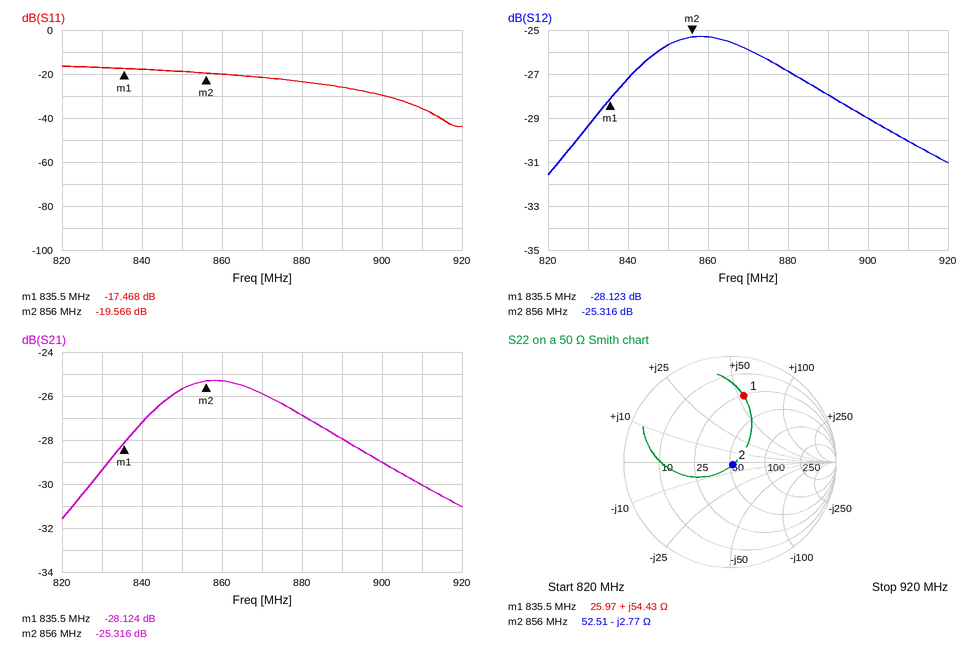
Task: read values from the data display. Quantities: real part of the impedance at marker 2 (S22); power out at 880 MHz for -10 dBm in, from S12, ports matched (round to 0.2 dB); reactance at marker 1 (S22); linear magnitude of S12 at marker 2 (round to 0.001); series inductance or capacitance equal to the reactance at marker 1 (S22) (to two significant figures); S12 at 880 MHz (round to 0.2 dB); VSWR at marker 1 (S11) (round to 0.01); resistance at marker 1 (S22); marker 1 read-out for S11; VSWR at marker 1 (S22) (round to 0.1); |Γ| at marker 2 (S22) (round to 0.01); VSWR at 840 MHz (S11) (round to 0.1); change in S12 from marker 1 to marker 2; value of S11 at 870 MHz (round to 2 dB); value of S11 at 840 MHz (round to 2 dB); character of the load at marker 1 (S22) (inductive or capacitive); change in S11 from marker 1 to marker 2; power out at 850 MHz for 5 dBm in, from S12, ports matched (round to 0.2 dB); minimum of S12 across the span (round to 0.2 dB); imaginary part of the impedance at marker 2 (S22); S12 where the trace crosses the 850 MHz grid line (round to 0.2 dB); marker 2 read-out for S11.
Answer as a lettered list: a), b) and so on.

a) 52.51 Ω
b) -36.8 dBm
c) +54.43 Ω
d) 0.054
e) 10 nH
f) -26.8 dB
g) 1.31
h) 25.97 Ω
i) -17.468 dB
j) 4.5
k) 0.04
l) 1.3
m) 2.807 dB
n) -22 dB
o) -18 dB
p) inductive
q) -2.098 dB
r) -20.6 dBm
s) -31.6 dB
t) -2.77 Ω
u) -25.6 dB
v) -19.566 dB
